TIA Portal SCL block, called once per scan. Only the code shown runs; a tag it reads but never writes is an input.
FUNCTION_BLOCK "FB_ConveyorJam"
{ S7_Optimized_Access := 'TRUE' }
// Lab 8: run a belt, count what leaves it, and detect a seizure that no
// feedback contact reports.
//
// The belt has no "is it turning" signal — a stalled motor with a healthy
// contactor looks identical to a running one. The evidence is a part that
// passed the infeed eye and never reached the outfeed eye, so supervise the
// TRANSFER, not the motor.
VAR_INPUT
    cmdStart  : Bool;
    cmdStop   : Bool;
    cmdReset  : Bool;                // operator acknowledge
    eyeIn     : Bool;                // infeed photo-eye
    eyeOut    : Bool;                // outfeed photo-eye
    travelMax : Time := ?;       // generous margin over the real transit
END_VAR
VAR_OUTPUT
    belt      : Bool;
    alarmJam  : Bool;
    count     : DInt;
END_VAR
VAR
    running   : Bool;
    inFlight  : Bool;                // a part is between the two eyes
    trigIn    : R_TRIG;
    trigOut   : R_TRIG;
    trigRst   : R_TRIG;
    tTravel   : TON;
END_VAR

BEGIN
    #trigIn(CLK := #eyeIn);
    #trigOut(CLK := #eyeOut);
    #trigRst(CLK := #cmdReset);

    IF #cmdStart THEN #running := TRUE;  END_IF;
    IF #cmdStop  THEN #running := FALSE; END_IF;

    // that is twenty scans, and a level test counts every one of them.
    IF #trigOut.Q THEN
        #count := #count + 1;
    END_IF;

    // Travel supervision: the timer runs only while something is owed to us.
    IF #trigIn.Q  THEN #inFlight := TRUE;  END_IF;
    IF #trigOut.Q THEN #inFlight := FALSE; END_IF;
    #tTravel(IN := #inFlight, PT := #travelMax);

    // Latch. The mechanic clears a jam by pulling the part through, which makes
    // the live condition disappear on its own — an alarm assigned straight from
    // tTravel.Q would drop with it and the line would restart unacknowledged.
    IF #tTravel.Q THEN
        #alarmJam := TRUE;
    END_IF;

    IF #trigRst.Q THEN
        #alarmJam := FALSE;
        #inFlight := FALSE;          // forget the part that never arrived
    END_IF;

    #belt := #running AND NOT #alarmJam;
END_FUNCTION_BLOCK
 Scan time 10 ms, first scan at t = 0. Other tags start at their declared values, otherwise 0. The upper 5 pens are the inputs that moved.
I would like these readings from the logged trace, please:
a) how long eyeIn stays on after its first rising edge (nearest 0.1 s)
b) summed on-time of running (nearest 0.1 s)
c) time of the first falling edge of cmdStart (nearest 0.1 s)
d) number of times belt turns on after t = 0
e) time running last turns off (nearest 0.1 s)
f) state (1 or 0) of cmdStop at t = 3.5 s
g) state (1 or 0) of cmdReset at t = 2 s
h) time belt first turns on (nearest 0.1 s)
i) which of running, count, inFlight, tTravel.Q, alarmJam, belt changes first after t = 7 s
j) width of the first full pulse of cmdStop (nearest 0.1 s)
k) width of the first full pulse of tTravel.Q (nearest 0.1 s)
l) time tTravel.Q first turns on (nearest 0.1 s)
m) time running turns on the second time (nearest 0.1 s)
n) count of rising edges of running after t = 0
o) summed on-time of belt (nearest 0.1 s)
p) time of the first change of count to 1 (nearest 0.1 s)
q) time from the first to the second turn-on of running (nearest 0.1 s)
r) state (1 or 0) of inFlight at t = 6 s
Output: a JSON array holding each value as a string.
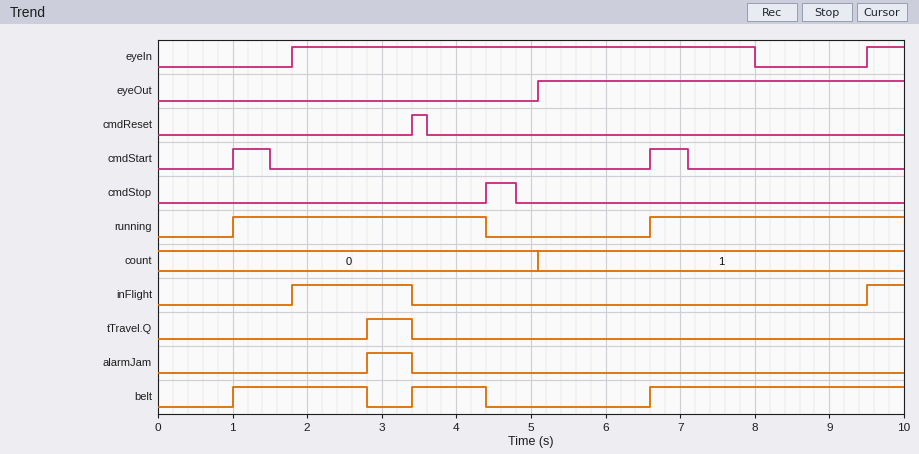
["6.2 s", "6.8 s", "1.5 s", "3", "4.4 s", "0", "0", "1.0 s", "inFlight", "0.4 s", "0.6 s", "2.8 s", "6.6 s", "2", "6.2 s", "5.1 s", "5.6 s", "0"]
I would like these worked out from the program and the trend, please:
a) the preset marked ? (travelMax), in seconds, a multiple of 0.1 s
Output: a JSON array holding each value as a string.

["1.0 s"]
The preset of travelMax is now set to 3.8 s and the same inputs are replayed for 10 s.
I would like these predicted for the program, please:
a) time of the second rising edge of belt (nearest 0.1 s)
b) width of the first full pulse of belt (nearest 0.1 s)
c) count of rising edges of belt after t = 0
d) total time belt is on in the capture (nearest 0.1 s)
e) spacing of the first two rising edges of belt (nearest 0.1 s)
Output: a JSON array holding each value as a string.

["6.6 s", "3.4 s", "2", "6.8 s", "5.6 s"]
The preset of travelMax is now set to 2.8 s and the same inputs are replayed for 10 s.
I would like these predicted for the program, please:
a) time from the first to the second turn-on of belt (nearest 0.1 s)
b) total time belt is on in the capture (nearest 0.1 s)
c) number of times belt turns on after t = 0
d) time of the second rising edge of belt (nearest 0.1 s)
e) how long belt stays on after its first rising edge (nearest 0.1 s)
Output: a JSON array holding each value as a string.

["5.6 s", "6.8 s", "2", "6.6 s", "3.4 s"]
